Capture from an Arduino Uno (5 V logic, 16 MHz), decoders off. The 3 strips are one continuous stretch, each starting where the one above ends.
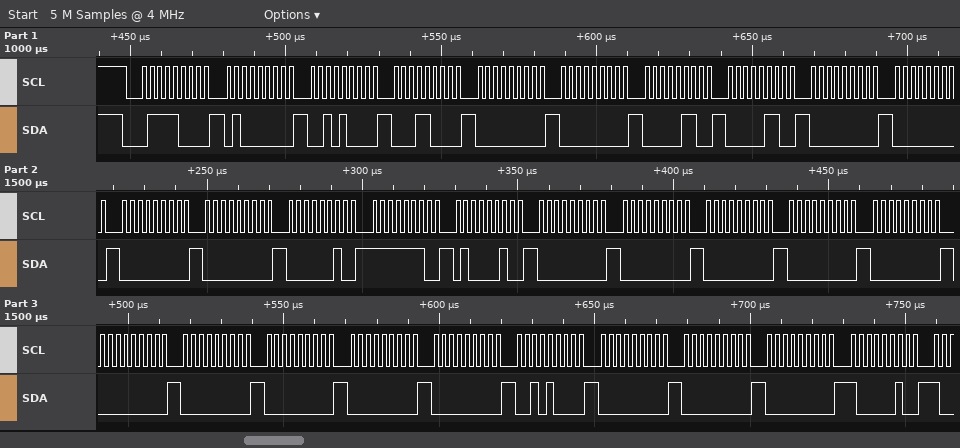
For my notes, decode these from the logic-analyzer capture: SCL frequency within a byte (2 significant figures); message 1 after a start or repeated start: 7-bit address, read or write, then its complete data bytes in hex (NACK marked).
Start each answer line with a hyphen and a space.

- 400 kHz
- 0x3C write: 40 28 18 00 00 06 06 00 00 00 00 02 FE 42 00 00 00 00 00 00 00 00 00 00 28 00 00 00 82
